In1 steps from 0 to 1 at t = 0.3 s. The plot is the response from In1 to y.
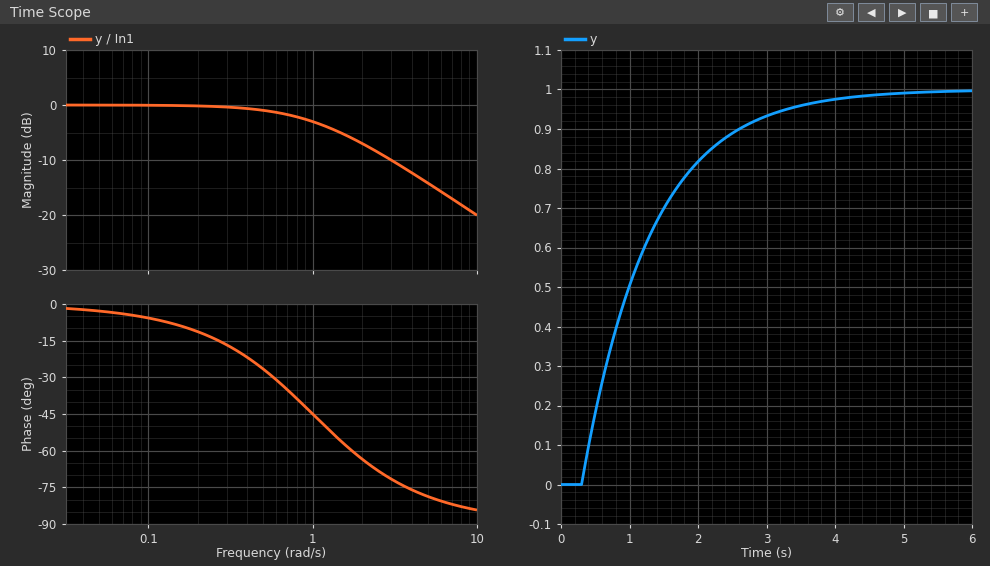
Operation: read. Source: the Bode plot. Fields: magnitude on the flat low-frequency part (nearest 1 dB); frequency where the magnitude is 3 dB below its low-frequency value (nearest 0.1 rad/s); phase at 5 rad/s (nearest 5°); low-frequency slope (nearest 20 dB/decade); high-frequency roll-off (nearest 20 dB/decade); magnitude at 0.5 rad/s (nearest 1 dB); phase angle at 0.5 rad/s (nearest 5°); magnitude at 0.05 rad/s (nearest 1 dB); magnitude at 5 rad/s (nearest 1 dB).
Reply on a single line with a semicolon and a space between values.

0 dB; 1.0 rad/s; -80°; 0 dB/decade; -20 dB/decade; -1 dB; -25°; 0 dB; -14 dB
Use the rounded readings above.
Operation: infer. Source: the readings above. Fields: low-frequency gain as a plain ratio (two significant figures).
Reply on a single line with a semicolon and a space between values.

1.0
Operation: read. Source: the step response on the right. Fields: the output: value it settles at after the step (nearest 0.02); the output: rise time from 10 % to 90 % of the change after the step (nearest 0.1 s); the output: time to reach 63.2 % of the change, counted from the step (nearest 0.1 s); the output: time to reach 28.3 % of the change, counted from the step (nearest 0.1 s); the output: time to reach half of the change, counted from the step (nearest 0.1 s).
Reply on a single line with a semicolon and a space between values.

1.00; 2.2 s; 1.0 s; 0.3 s; 0.7 s
